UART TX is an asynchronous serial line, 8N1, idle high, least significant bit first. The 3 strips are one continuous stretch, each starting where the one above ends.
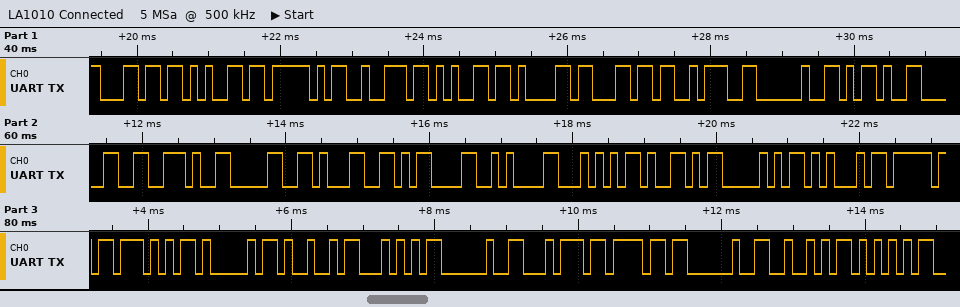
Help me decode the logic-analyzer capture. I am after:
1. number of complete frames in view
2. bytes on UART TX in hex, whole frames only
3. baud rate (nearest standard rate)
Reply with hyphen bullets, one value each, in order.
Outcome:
- 31
- 6C 65 5F 72 65 61 6C 3A 20 2D 30 2E 30 31 0D 0A 54 59 50 45 5F 57 41 49 54 20 74 6F 20 52 55
- 9600 baud
